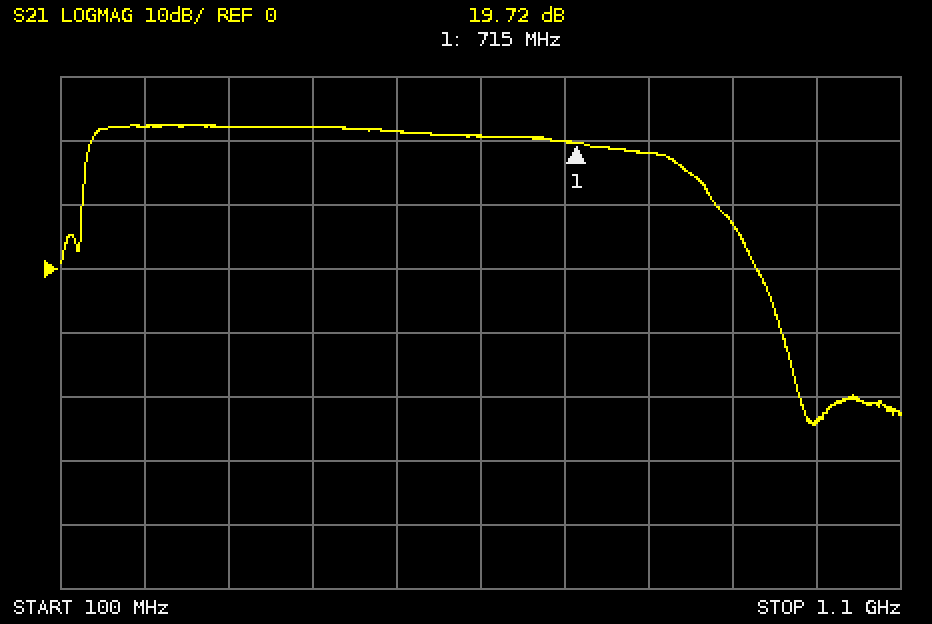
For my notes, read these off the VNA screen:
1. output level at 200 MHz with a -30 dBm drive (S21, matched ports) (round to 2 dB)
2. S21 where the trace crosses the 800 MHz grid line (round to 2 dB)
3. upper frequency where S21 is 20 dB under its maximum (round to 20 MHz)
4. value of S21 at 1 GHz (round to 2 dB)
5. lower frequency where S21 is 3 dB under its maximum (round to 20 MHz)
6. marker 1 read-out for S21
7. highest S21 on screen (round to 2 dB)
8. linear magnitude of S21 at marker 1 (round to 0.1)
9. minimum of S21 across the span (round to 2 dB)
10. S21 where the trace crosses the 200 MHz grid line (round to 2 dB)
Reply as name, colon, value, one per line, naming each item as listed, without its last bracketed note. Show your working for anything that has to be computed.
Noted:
output level at 200 MHz with a -30 dBm drive (S21, matched ports): -30 dBm + (22 dB) = -8 dBm
S21 where the trace crosses the 800 MHz grid line: 18 dB
upper frequency where S21 is 20 dB under its maximum: 920 MHz
value of S21 at 1 GHz: -24 dB
lower frequency where S21 is 3 dB under its maximum: 140 MHz
marker 1 read-out for S21: 19.72 dB
highest S21 on screen: 22 dB
linear magnitude of S21 at marker 1: 10^(19.72/20) ≈ 9.7
minimum of S21 across the span: -24 dB
S21 where the trace crosses the 200 MHz grid line: 22 dB
